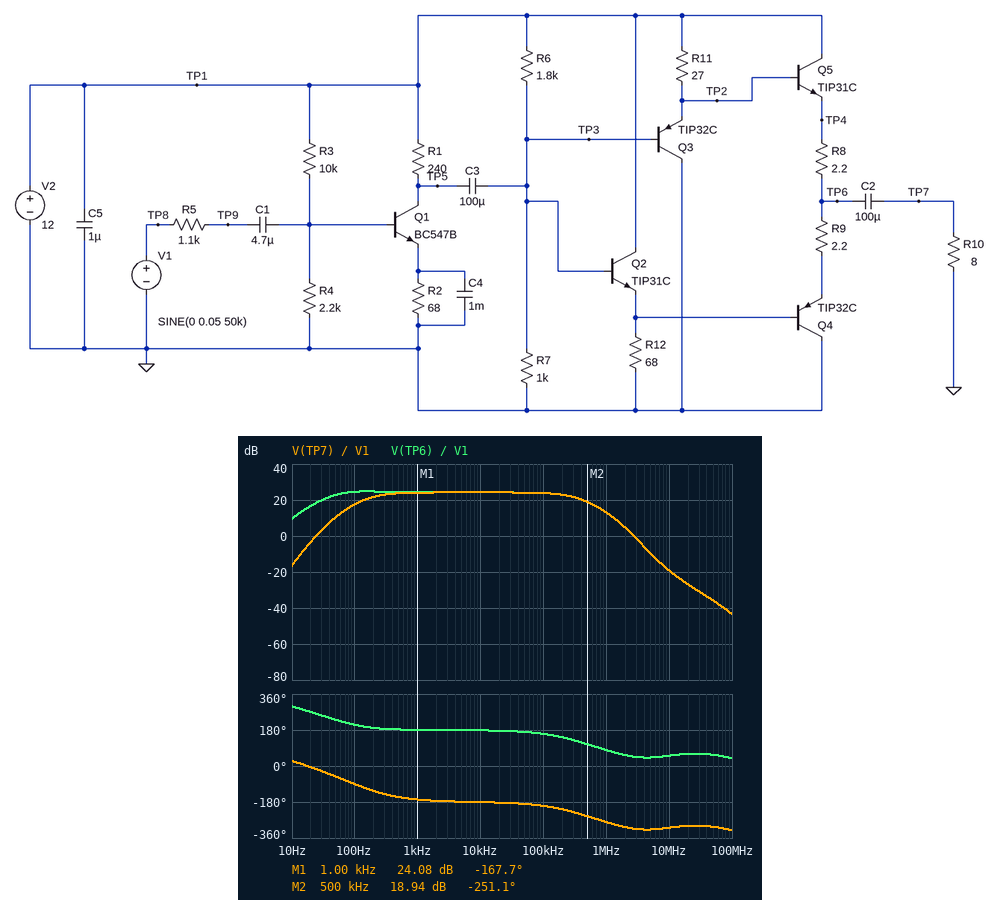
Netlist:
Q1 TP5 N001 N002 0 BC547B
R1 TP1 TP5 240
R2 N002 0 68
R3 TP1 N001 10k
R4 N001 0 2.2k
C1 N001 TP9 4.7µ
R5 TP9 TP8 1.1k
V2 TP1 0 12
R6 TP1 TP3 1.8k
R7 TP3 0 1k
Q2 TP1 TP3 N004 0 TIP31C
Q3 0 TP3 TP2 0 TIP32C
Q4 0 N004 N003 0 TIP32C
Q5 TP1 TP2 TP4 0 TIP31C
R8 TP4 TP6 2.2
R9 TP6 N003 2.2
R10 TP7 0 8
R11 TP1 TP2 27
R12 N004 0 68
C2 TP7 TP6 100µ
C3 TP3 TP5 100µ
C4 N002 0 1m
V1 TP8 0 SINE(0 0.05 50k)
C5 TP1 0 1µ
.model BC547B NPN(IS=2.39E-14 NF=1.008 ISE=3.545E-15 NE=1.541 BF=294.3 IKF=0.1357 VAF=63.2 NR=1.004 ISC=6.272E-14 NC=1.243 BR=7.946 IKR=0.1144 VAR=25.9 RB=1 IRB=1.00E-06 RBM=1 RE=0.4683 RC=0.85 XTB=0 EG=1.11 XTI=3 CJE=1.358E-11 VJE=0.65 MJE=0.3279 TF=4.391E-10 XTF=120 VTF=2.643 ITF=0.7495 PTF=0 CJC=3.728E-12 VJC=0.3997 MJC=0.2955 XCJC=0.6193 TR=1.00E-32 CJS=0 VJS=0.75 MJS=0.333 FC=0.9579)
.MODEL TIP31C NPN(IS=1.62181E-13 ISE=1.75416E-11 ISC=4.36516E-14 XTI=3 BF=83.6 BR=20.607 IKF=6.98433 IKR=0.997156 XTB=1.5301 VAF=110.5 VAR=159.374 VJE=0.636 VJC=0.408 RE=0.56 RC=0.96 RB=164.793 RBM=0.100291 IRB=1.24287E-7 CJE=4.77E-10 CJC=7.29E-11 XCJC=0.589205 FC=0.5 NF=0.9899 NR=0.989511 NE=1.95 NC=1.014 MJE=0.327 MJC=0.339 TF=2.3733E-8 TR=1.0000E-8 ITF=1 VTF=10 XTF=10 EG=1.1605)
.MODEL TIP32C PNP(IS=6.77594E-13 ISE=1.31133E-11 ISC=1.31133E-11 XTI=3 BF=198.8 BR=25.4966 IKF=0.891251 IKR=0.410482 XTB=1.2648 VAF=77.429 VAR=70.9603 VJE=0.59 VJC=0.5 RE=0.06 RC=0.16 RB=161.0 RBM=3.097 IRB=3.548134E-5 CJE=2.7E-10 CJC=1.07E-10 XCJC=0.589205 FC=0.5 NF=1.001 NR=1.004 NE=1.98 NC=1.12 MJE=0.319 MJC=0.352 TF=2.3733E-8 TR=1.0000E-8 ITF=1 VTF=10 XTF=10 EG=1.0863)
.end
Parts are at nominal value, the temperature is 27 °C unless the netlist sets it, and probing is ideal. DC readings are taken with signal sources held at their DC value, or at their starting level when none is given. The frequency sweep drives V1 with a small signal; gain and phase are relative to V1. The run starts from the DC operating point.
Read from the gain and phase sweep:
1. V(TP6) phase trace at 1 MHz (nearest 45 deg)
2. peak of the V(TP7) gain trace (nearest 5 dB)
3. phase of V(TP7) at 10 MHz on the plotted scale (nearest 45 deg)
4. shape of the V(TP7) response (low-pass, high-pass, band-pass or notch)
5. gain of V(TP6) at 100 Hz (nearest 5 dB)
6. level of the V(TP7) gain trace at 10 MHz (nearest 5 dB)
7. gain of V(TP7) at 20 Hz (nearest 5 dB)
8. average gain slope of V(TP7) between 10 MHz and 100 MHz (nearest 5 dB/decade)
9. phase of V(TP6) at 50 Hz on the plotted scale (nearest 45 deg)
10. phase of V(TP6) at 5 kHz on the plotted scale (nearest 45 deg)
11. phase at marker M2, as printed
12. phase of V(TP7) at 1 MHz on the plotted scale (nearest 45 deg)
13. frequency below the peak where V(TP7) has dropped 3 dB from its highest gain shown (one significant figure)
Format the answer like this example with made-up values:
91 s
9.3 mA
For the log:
90 deg
25 dB
-315 deg
band-pass
25 dB
-20 dB
-5 dB
-25 dB/decade
225 deg
180 deg
-251.1 deg
-270 deg
200 Hz
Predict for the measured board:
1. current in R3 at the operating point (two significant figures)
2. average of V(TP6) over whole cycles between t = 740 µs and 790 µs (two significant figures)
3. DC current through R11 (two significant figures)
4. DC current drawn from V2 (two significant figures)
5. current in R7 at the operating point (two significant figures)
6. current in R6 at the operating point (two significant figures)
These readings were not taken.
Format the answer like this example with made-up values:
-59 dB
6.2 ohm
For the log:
1.0 mA
4.8 V
240 mA
350 mA
4.8 mA
4.0 mA
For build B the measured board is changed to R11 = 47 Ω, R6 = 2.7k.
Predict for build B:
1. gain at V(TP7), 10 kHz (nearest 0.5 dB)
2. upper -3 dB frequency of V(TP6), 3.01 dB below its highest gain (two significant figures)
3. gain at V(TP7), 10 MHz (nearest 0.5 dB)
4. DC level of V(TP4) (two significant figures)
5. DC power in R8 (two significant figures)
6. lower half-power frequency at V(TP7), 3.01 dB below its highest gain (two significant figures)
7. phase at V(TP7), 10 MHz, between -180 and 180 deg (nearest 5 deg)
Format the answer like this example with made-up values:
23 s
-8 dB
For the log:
24.5 dB
450 kHz
-18.0 dB
3.6 V
1.2 mW
170 Hz
45 deg
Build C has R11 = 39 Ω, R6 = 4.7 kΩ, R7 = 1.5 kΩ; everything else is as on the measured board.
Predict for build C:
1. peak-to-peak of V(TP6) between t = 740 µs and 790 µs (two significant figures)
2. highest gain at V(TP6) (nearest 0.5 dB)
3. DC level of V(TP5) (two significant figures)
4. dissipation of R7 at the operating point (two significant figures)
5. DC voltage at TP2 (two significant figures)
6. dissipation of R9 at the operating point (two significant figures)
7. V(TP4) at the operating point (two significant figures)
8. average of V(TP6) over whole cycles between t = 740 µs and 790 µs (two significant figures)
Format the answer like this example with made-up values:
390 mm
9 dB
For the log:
1.7 V
26.0 dB
7.4 V
8.9 mW
4.4 V
1.4 mW
3.7 V
3.6 V
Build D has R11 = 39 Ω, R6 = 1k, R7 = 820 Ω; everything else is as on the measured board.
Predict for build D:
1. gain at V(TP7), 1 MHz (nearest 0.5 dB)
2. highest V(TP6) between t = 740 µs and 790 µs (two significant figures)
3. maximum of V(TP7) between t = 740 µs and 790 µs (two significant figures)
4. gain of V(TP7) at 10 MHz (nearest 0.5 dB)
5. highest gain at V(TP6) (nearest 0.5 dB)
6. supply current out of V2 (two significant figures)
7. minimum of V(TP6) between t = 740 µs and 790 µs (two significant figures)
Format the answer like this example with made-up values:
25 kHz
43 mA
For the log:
16.5 dB
6.1 V
700 mV
-18.5 dB
24.0 dB
270 mA
4.7 V
